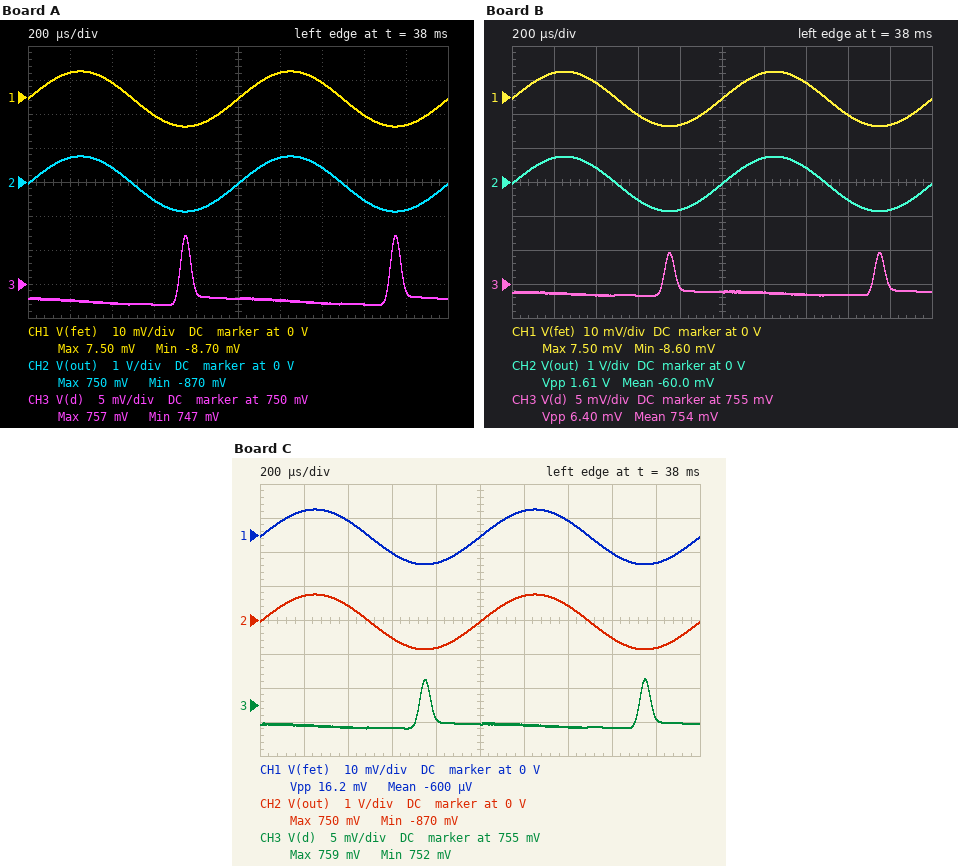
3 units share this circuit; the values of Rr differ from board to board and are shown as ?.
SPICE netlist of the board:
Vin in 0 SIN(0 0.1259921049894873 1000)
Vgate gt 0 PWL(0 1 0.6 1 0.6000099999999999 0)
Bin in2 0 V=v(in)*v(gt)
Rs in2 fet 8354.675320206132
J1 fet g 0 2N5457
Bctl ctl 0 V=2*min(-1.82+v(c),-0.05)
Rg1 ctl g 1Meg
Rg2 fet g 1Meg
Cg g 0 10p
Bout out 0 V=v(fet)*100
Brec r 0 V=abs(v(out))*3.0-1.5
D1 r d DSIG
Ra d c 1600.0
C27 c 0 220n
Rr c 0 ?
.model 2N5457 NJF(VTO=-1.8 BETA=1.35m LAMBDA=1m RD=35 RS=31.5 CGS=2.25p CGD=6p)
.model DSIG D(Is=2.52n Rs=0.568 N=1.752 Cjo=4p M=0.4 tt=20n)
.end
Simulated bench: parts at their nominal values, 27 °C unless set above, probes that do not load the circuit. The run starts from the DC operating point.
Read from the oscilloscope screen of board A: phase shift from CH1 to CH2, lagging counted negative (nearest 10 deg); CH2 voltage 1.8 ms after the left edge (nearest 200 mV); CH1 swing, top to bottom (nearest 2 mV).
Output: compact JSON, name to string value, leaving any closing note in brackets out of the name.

{"phase shift from CH1 to CH2, lagging counted negative": "0 deg", "CH2 voltage 1.8 ms after the left edge": "-800 mV", "CH1 swing, top to bottom": "16 mV"}
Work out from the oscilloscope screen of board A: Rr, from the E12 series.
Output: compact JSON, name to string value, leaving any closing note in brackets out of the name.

{"Rr, from the E12 series": "2.2 MΩ"}
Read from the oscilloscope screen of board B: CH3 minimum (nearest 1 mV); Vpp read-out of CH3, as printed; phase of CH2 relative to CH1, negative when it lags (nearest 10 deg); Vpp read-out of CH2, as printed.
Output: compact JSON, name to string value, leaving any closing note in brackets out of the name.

{"CH3 minimum": "753 mV", "Vpp read-out of CH3, as printed": "6.40 mV", "phase of CH2 relative to CH1, negative when it lags": "0 deg", "Vpp read-out of CH2, as printed": "1.61 V"}
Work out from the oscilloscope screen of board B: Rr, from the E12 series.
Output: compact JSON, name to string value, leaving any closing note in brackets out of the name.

{"Rr, from the E12 series": "3.9 MΩ"}
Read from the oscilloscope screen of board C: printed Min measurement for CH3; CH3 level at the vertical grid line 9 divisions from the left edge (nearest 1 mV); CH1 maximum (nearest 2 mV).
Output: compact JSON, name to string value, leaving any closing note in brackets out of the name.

{"printed Min measurement for CH3": "752 mV", "CH3 level at the vertical grid line 9 divisions from the left edge": "753 mV", "CH1 maximum": "8 mV"}
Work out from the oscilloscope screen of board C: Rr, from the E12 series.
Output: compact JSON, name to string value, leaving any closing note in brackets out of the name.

{"Rr, from the E12 series": "3.3 MΩ"}
